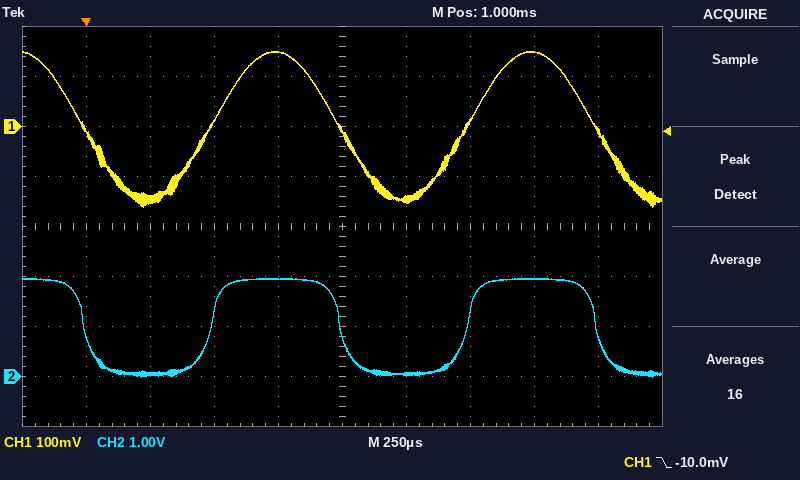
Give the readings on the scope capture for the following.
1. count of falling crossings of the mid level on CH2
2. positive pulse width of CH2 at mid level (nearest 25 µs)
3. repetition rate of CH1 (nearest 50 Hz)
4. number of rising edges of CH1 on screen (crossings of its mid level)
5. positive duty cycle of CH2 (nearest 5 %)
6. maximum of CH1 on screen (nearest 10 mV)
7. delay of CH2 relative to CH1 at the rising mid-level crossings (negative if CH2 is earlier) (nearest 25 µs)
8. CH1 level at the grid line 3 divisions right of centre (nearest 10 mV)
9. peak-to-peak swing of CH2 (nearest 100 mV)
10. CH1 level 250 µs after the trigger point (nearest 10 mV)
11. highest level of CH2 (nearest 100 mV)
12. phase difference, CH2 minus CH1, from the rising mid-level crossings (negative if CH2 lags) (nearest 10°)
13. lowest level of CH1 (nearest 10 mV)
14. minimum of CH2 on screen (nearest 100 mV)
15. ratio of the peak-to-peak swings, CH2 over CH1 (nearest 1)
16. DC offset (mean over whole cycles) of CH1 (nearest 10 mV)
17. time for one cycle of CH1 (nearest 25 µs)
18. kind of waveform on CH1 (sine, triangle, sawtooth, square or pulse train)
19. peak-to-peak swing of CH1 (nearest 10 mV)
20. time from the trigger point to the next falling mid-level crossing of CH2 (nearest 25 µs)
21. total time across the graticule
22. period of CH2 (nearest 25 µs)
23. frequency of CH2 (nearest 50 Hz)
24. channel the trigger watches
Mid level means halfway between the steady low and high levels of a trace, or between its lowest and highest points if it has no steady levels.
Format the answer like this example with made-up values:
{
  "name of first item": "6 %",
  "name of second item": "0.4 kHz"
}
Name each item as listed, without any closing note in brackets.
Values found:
{
  "count of falling crossings of the mid level on CH2": "3",
  "positive pulse width of CH2 at mid level": "500 µs",
  "repetition rate of CH1": "1.00 kHz",
  "number of rising edges of CH1 on screen": "2",
  "positive duty cycle of CH2": "50 %",
  "maximum of CH1 on screen": "150 mV",
  "delay of CH2 relative to CH1 at the rising mid-level crossings (negative if CH2 is earlier)": "0 µs",
  "CH1 level at the grid line 3 divisions right of centre": "150 mV",
  "peak-to-peak swing of CH2": "2.0 V",
  "CH1 level 250 µs after the trigger point": "-150 mV",
  "highest level of CH2": "2.0 V",
  "phase difference, CH2 minus CH1, from the rising mid-level crossings (negative if CH2 lags)": "0°",
  "lowest level of CH1": "-160 mV",
  "minimum of CH2 on screen": "0.0 V",
  "ratio of the peak-to-peak swings, CH2 over CH1": "6",
  "DC offset (mean over whole cycles) of CH1": "0 mV",
  "time for one cycle of CH1": "1.000 ms",
  "kind of waveform on CH1": "sine",
  "peak-to-peak swing of CH1": "310 mV",
  "time from the trigger point to the next falling mid-level crossing of CH2": "1.000 ms",
  "total time across the graticule": "2.5 ms",
  "period of CH2": "1.000 ms",
  "frequency of CH2": "1.00 kHz",
  "channel the trigger watches": "CH1"
}
